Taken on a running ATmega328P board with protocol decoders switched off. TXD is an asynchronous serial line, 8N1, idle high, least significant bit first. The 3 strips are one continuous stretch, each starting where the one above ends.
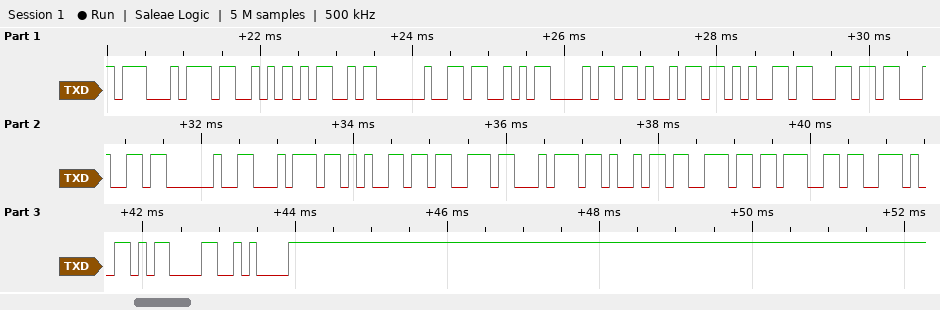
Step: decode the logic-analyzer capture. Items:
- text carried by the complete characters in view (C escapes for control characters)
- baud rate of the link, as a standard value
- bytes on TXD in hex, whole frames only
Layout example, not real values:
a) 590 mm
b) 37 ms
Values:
a) "GSM Shield testing.\r\n"
b) 9600 baud
c) 47 53 4D 20 53 68 69 65 6C 64 20 74 65 73 74 69 6E 67 2E 0D 0A
